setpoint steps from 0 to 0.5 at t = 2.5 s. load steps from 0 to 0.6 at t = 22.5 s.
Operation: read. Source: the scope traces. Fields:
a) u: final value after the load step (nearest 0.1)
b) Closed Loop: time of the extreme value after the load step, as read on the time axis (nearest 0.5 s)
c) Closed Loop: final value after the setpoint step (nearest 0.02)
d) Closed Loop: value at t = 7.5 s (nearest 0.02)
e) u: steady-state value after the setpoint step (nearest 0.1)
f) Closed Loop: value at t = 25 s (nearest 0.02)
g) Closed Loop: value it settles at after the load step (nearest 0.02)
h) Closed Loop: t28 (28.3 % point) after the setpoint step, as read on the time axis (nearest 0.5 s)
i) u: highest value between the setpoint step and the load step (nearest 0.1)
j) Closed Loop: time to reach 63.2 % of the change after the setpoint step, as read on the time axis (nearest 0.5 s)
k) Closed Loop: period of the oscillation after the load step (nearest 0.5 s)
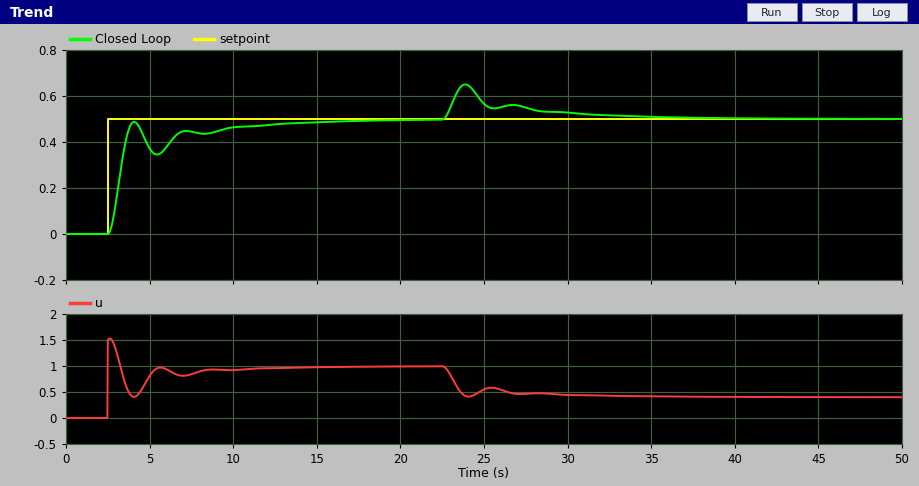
0.4
24.0 s
0.50
0.44
1.0
0.56
0.50
3.0 s
1.5
3.5 s
3.0 s
